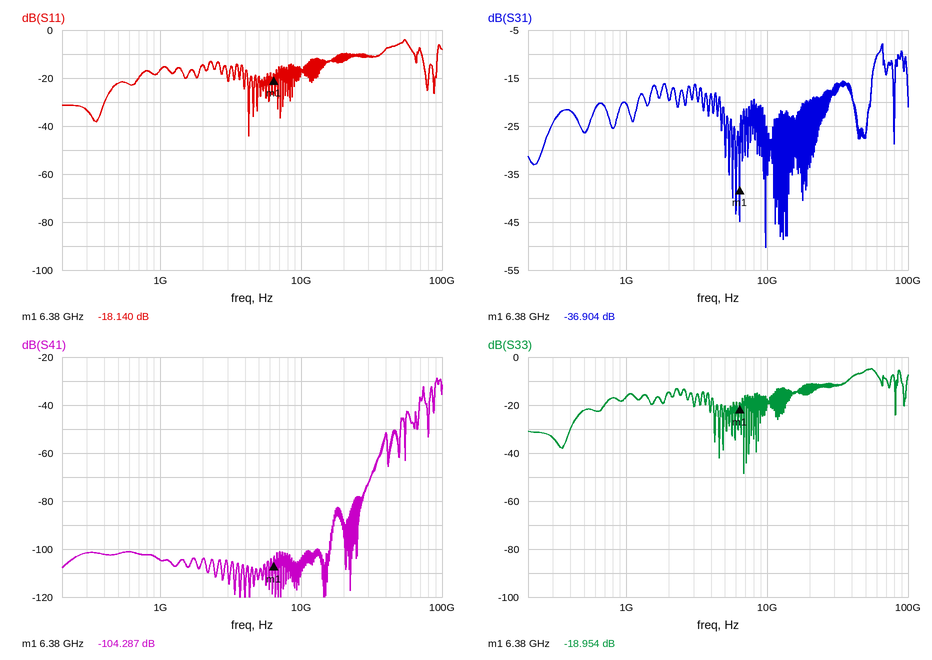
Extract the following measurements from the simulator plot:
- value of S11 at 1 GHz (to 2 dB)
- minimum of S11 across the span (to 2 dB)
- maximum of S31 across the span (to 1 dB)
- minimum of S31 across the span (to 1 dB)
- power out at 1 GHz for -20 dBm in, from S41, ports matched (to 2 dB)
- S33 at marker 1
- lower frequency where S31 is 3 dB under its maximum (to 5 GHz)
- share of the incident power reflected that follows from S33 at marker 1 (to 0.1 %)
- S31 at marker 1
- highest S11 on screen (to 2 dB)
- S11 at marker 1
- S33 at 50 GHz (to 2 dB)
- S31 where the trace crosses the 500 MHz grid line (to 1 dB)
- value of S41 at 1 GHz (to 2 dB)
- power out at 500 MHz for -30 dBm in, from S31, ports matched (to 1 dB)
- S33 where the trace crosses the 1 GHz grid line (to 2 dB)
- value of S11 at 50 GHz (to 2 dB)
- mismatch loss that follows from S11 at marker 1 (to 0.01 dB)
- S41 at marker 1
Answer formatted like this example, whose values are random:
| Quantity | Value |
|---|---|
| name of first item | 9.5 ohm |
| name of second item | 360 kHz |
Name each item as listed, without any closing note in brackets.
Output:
| Quantity | Value |
|---|---|
| value of S11 at 1 GHz | -16 dB |
| minimum of S11 across the span | -44 dB |
| maximum of S31 across the span | -8 dB |
| minimum of S31 across the span | -50 dB |
| power out at 1 GHz for -20 dBm in, from S41, ports matched | -124 dBm |
| S33 at marker 1 | -18.954 dB |
| lower frequency where S31 is 3 dB under its maximum | 60 GHz |
| share of the incident power reflected that follows from S33 at marker 1 | 1.3 % |
| S31 at marker 1 | -36.904 dB |
| highest S11 on screen | -4 dB |
| S11 at marker 1 | -18.140 dB |
| S33 at 50 GHz | -6 dB |
| S31 where the trace crosses the 500 MHz grid line | -26 dB |
| value of S41 at 1 GHz | -104 dB |
| power out at 500 MHz for -30 dBm in, from S31, ports matched | -56 dBm |
| S33 where the trace crosses the 1 GHz grid line | -16 dB |
| value of S11 at 50 GHz | -6 dB |
| mismatch loss that follows from S11 at marker 1 | 0.07 dB |
| S41 at marker 1 | -104.287 dB |
